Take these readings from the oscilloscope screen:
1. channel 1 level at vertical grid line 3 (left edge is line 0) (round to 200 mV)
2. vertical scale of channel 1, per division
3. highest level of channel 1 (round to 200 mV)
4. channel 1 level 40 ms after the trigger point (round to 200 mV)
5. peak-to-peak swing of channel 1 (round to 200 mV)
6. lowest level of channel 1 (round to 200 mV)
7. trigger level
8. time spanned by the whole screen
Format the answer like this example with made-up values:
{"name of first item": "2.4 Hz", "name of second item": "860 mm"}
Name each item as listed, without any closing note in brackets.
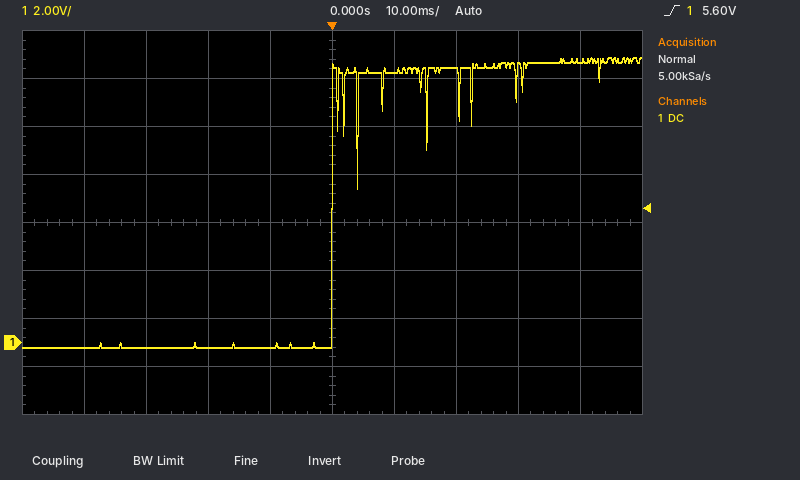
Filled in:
{"channel 1 level at vertical grid line 3 (left edge is line 0)": "-200 mV", "vertical scale of channel 1, per division": "2 V", "highest level of channel 1": "11.8 V", "channel 1 level 40 ms after the trigger point": "11.8 V", "peak-to-peak swing of channel 1": "12.0 V", "lowest level of channel 1": "-200 mV", "trigger level": "5.60 V", "time spanned by the whole screen": "100 ms"}
